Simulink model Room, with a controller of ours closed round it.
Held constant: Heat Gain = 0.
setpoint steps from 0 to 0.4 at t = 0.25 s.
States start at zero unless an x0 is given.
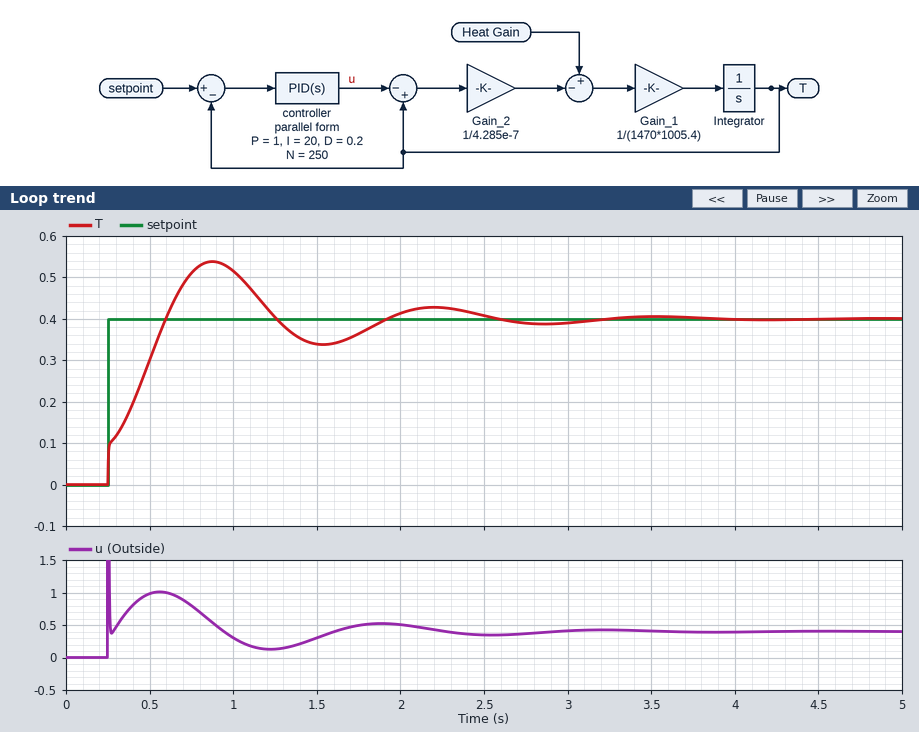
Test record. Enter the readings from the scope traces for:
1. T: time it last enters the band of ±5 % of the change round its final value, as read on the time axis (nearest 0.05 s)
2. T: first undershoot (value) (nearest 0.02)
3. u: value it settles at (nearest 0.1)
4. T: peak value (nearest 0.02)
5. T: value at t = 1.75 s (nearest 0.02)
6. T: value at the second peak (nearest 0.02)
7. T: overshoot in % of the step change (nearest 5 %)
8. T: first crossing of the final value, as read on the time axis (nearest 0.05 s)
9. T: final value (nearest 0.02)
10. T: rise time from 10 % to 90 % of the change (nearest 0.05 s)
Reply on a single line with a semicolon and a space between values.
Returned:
2.35 s; 0.34; 0.4; 0.54; 0.36; 0.42; 35 %; 0.60 s; 0.40; 0.30 s
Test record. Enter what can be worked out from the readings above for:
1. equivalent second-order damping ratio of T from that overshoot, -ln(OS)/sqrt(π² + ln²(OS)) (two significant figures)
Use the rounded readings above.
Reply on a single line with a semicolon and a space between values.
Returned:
0.32
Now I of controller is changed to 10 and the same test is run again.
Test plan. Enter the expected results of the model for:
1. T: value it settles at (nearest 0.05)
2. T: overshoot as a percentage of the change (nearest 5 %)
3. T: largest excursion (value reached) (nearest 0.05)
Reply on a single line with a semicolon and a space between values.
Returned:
0.40; 25 %; 0.50
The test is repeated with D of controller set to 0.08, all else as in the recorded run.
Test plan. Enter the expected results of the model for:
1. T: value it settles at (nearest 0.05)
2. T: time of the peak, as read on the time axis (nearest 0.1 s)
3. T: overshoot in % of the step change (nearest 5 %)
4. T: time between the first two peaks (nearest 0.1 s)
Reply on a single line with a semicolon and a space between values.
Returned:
0.40; 0.8 s; 40 %; 1.2 s
